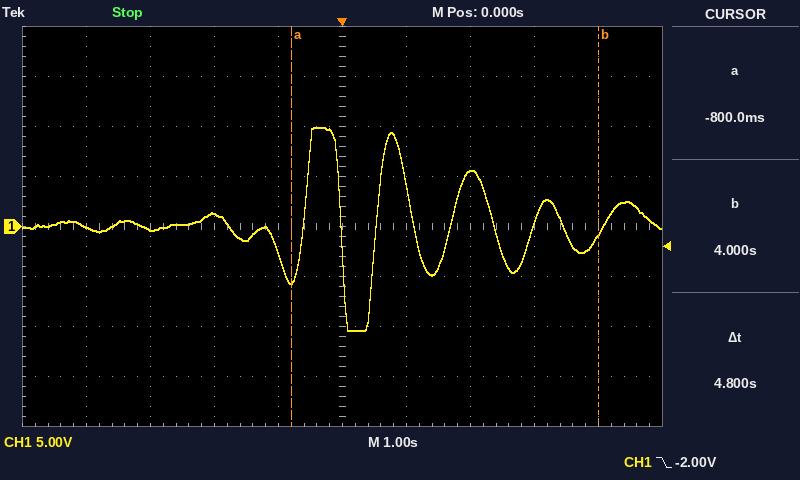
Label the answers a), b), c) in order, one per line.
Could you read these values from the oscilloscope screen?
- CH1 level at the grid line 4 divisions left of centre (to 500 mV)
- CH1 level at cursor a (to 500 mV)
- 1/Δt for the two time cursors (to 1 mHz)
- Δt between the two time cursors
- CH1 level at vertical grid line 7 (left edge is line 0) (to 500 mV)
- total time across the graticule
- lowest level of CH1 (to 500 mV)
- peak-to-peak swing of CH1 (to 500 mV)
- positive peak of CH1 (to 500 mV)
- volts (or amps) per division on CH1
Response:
a) 0.0 V
b) -5.5 V
c) 208 mHz
d) 4.8 s
e) 5.5 V
f) 10 s
g) -10.5 V
h) 20.5 V
i) 10.0 V
j) 5 V
